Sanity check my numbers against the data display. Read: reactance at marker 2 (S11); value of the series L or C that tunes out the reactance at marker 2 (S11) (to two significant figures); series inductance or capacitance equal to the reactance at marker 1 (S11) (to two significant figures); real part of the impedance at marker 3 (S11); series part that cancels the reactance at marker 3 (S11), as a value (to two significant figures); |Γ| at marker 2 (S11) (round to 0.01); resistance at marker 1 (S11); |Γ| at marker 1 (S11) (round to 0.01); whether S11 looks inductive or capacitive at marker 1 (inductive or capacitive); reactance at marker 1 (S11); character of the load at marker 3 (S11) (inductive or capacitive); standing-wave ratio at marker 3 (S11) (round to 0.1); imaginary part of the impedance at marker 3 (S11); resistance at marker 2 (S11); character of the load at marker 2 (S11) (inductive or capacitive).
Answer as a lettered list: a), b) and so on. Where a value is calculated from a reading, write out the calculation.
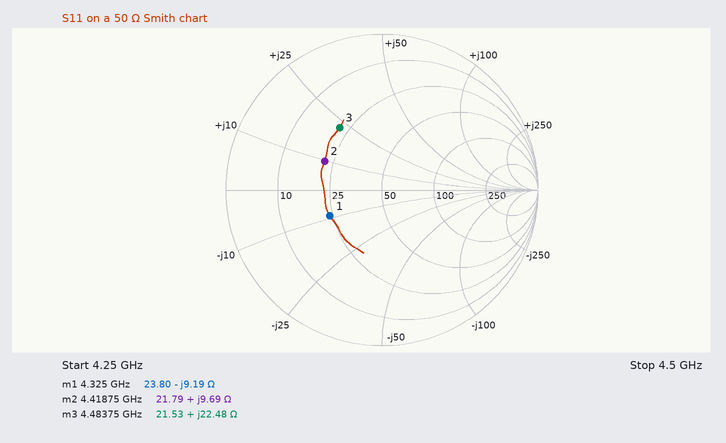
a) +9.69 Ω
b) C = 1/(2π × 4.41875 GHz × 9.69 Ω) ≈ 3.7 pF
c) C = 1/(2π × 4.325 GHz × 9.19 Ω) ≈ 4.0 pF
d) 21.53 Ω
e) C = 1/(2π × 4.48375 GHz × 22.48 Ω) ≈ 1.6 pF
f) 0.41
g) 23.80 Ω
h) 0.37
i) capacitive
j) -9.19 Ω
k) inductive
l) 2.9
m) +22.48 Ω
n) 21.79 Ω
o) inductive
